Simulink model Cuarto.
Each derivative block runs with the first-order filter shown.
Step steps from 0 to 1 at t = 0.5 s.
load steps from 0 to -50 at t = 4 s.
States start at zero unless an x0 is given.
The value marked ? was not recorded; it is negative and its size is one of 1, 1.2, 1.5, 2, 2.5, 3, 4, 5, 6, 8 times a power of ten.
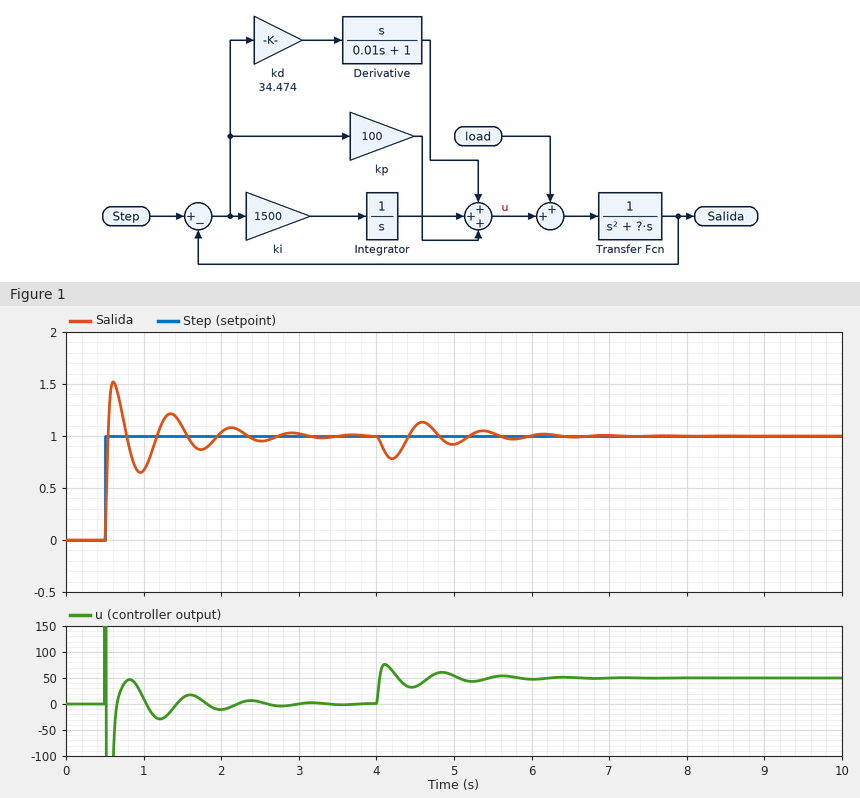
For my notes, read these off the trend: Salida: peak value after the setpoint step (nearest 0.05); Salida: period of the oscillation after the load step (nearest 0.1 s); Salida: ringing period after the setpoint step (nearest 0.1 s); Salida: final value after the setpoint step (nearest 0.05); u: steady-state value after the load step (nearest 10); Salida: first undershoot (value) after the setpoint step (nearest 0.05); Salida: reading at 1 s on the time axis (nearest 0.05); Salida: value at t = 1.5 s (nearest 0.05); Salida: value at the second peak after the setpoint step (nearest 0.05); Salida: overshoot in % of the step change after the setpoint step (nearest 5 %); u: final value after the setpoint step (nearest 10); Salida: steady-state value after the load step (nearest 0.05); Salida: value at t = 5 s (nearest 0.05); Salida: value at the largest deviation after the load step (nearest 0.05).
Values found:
1.50
0.8 s
0.7 s
1.00
50
0.65
0.65
1.10
1.20
50 %
0
1.00
0.90
0.80
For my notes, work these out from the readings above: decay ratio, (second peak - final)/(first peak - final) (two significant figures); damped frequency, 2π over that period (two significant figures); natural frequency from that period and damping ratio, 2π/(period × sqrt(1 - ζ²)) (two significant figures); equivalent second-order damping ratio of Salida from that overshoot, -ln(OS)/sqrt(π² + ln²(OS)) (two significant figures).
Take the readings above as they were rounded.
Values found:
0.40
9.0 rad/s
9.2 rad/s
0.22
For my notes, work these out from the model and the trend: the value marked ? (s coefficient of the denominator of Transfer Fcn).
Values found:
-10
